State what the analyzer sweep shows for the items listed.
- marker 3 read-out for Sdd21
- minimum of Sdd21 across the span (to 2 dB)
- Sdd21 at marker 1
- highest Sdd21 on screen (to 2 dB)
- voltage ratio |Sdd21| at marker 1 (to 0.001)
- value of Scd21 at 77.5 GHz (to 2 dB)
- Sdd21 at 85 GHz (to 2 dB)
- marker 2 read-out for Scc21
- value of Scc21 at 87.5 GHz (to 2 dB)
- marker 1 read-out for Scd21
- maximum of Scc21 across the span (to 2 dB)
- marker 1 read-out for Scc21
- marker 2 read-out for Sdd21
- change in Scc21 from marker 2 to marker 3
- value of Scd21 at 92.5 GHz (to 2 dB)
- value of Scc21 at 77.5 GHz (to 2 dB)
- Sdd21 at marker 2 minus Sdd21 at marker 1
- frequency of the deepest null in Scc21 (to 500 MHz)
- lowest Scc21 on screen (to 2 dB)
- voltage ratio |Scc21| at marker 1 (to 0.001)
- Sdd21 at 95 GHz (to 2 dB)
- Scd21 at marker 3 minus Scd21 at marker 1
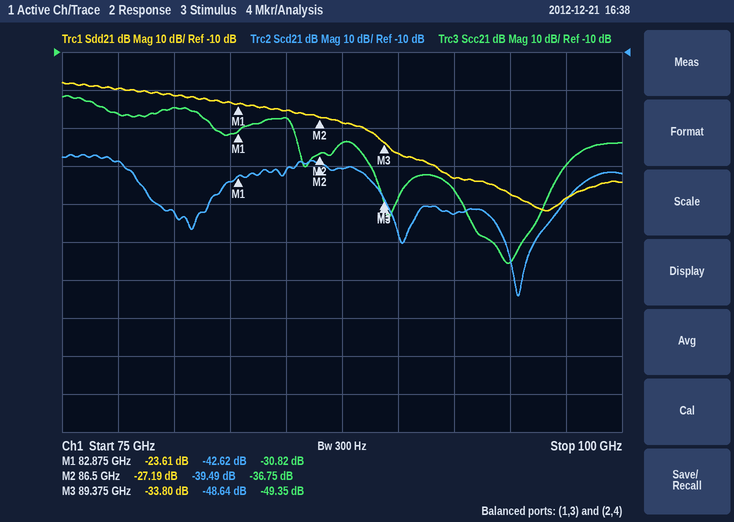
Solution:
-33.80 dB
-52 dB
-23.61 dB
-18 dB
0.066
-38 dB
-26 dB
-36.75 dB
-34 dB
-42.62 dB
-22 dB
-30.82 dB
-27.19 dB
-12.60 dB
-52 dB
-26 dB
-3.58 dB
95.0 GHz
-66 dB
0.029
-48 dB
-6.02 dB
